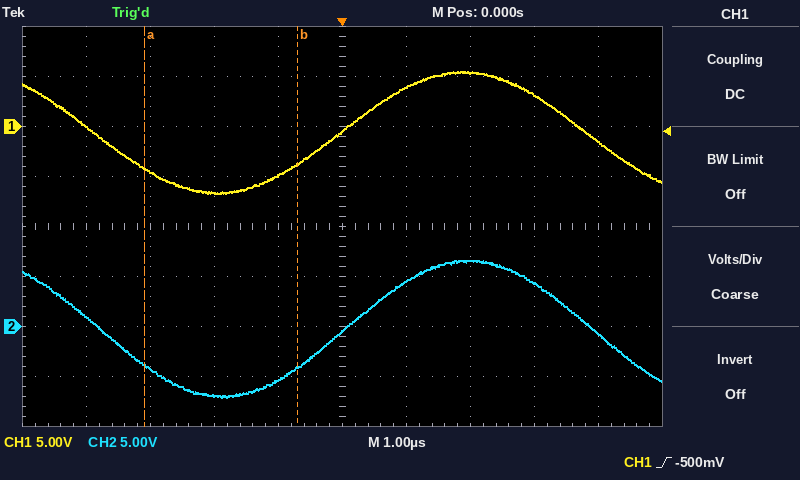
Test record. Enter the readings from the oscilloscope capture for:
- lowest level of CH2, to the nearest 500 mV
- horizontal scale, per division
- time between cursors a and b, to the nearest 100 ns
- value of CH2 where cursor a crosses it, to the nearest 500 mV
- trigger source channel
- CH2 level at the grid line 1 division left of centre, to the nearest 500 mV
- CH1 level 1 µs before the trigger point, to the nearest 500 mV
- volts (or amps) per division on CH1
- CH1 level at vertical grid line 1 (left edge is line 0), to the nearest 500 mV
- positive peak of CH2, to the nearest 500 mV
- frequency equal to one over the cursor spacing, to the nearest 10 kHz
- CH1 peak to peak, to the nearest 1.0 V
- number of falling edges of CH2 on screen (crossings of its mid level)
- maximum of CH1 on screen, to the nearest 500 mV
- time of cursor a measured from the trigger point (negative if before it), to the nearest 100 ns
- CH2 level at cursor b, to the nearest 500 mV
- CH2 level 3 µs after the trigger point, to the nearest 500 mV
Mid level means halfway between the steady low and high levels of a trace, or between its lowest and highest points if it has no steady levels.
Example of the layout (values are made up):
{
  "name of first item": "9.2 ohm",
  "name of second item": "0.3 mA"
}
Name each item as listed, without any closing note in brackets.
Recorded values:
{
  "lowest level of CH2, to the nearest 500 mV": "-7.0 V",
  "horizontal scale, per division": "1 µs",
  "time between cursors a and b, to the nearest 100 ns": "2.4 µs",
  "value of CH2 where cursor a crosses it, to the nearest 500 mV": "-4.0 V",
  "trigger source channel": "CH1",
  "CH2 level at the grid line 1 division left of centre, to the nearest 500 mV": "-5.5 V",
  "CH1 level 1 µs before the trigger point, to the nearest 500 mV": "-5.0 V",
  "volts (or amps) per division on CH1": "5 V",
  "CH1 level at vertical grid line 1 (left edge is line 0), to the nearest 500 mV": "0.0 V",
  "positive peak of CH2, to the nearest 500 mV": "6.5 V",
  "frequency equal to one over the cursor spacing, to the nearest 10 kHz": "420 kHz",
  "CH1 peak to peak, to the nearest 1.0 V": "12.0 V",
  "number of falling edges of CH2 on screen": "2",
  "maximum of CH1 on screen, to the nearest 500 mV": "5.5 V",
  "time of cursor a measured from the trigger point (negative if before it), to the nearest 100 ns": "-3.1 µs",
  "CH2 level at cursor b, to the nearest 500 mV": "-4.0 V",
  "CH2 level 3 µs after the trigger point, to the nearest 500 mV": "4.5 V"
}
